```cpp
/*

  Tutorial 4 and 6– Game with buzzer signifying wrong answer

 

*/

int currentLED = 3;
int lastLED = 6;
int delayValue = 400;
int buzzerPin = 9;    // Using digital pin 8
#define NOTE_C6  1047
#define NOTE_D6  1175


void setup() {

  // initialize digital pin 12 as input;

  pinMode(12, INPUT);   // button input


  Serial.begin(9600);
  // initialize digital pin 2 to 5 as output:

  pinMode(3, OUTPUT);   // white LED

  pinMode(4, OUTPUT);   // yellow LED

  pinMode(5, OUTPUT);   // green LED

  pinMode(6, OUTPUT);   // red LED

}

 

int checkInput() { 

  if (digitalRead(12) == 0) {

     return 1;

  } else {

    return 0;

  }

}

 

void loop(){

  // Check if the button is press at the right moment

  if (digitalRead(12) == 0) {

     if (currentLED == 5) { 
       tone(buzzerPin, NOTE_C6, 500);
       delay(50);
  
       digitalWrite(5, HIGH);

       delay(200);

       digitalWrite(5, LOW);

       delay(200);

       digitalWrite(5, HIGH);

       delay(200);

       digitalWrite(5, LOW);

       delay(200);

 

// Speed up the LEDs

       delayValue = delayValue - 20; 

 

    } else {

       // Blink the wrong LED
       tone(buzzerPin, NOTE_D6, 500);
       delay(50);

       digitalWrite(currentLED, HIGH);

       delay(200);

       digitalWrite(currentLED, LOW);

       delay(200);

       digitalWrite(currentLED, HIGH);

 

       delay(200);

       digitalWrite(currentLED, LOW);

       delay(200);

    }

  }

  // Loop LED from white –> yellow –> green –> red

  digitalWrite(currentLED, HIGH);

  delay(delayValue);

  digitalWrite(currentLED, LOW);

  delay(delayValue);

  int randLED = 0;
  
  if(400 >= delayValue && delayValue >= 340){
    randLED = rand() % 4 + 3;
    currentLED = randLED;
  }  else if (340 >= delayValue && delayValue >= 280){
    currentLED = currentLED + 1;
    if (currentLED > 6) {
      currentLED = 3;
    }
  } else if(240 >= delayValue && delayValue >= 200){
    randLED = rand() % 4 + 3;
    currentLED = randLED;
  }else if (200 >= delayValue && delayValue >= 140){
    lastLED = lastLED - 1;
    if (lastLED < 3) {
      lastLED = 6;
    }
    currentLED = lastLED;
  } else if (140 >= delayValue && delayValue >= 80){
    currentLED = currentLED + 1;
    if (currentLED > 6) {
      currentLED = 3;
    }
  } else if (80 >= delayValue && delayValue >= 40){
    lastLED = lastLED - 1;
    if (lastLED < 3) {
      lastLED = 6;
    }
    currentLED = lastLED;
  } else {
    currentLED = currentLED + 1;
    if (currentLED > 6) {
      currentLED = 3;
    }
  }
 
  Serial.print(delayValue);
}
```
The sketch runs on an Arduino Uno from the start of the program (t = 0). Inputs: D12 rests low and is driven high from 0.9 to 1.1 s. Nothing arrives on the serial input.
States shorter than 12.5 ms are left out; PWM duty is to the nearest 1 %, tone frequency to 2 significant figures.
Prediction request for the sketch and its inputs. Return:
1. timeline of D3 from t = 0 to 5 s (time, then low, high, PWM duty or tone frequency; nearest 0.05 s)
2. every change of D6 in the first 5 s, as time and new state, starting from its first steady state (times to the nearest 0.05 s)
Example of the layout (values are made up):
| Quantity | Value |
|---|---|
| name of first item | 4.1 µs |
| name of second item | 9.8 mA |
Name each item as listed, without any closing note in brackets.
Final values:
| Quantity | Value |
|---|---|
| timeline of D3 from t = 0 to 5 s | 0 s low; 0.05 s high; 0.25 s low; 0.45 s high; 0.65 s low; 0.85 s high; 1.25 s low |
| every change of D6 in the first 5 s, as time and new state, starting from its first steady state | 0 s low; 1.7 s high; 1.9 s low; 2.1 s high; 2.3 s low; 2.5 s high; 2.9 s low |
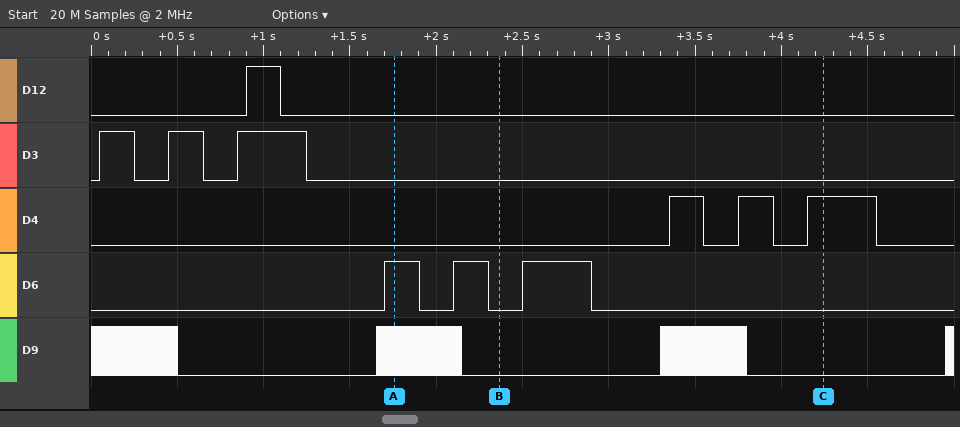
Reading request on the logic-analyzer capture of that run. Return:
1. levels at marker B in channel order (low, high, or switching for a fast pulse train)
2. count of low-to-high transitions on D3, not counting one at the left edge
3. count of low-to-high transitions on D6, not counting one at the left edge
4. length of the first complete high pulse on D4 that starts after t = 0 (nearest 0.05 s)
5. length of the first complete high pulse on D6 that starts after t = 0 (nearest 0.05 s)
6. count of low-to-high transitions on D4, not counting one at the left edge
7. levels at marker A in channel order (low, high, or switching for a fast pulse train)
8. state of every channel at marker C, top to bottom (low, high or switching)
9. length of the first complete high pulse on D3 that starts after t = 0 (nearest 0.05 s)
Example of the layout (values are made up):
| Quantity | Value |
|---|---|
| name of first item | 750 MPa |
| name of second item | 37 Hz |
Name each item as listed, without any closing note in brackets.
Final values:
| Quantity | Value |
|---|---|
| levels at marker B in channel order | D12 low, D3 low, D4 low, D6 low, D9 low |
| count of low-to-high transitions on D3, not counting one at the left edge | 3 |
| count of low-to-high transitions on D6, not counting one at the left edge | 3 |
| length of the first complete high pulse on D4 that starts after t = 0 | 0.20 s |
| length of the first complete high pulse on D6 that starts after t = 0 | 0.20 s |
| count of low-to-high transitions on D4, not counting one at the left edge | 3 |
| levels at marker A in channel order | D12 low, D3 low, D4 low, D6 high, D9 switching |
| state of every channel at marker C, top to bottom | D12 low, D3 low, D4 high, D6 low, D9 low |
| length of the first complete high pulse on D3 that starts after t = 0 | 0.20 s |
